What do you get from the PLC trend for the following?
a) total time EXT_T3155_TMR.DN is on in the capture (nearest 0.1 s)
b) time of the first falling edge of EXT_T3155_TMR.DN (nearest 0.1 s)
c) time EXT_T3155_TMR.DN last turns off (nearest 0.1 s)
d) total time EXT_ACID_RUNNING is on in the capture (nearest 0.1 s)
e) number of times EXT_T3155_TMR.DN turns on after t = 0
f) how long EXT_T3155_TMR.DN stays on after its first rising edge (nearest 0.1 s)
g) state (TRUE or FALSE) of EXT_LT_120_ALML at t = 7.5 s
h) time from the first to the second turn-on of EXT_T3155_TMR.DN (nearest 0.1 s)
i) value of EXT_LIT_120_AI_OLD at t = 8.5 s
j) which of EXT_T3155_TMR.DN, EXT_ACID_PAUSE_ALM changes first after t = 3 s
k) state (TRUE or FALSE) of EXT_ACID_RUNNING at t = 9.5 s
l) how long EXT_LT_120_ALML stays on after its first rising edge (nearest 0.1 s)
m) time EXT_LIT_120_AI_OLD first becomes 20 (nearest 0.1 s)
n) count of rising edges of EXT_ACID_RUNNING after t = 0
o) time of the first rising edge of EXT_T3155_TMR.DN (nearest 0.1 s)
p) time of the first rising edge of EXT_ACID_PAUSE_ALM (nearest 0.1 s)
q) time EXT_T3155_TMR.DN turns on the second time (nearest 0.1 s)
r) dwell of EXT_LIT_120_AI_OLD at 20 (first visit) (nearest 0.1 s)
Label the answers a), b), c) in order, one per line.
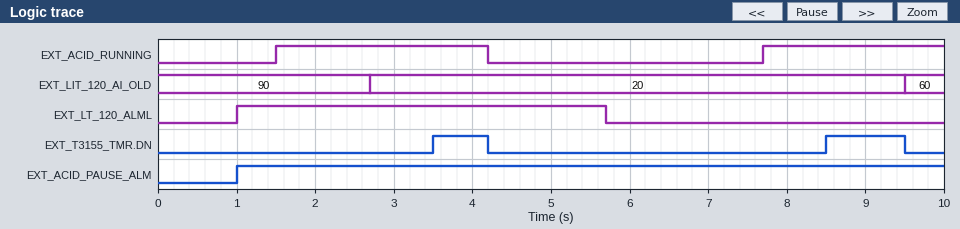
a) 1.7 s
b) 4.2 s
c) 9.5 s
d) 5.0 s
e) 2
f) 0.7 s
g) FALSE
h) 5.0 s
i) 20
j) EXT_T3155_TMR.DN
k) TRUE
l) 4.7 s
m) 2.7 s
n) 2
o) 3.5 s
p) 1.0 s
q) 8.5 s
r) 6.8 s
